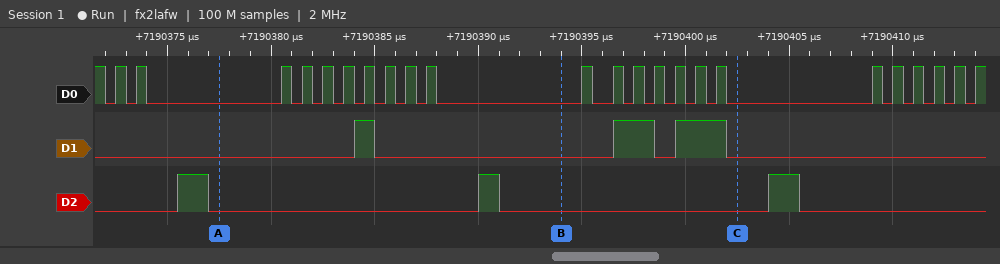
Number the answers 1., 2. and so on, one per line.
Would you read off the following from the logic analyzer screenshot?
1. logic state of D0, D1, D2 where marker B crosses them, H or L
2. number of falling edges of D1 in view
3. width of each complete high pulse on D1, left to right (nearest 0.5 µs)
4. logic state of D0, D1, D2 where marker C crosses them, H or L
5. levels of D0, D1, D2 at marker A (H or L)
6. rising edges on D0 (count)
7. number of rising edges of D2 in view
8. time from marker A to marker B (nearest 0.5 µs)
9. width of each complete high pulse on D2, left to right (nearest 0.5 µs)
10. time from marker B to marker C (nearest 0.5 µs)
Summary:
1. D0=L, D1=L, D2=L
2. 3
3. 1 µs, 2 µs, 2.5 µs
4. D0=L, D1=L, D2=L
5. D0=L, D1=L, D2=L
6. 23
7. 3
8. 16.5 µs
9. 1.5 µs, 1 µs, 1.5 µs
10. 8.5 µs
